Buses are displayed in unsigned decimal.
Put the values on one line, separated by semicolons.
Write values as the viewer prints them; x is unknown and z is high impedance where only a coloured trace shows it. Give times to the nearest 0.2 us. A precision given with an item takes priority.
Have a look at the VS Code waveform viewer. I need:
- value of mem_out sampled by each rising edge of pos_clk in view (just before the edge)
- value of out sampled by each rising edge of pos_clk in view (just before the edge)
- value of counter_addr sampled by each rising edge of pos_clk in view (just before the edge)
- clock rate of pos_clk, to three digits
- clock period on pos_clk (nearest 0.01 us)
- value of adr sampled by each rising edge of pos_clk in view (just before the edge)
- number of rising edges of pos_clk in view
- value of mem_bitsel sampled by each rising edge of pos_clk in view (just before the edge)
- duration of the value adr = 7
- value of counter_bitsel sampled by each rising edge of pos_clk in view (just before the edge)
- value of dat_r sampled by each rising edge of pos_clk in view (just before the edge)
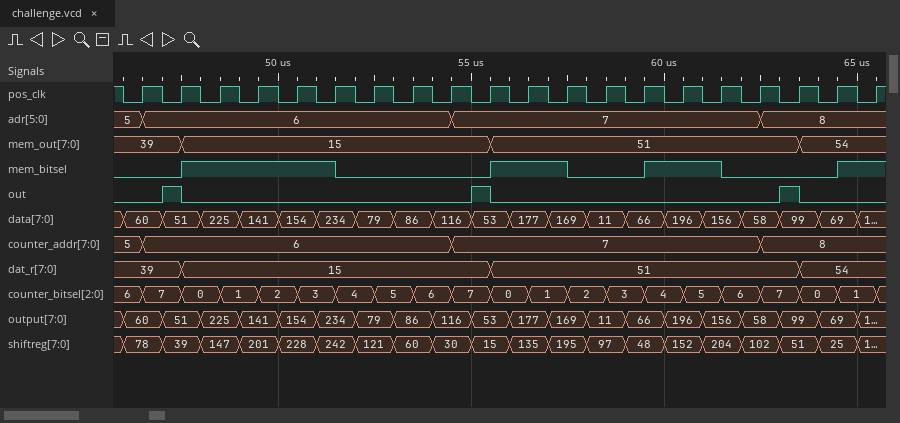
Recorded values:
39, 39, 15, 15, 15, 15, 15, 15, 15, 15, 51, 51, 51, 51, 51, 51, 51, 51, 54, 54; 0 1 0 0 0 0 0 0 0 1 0 0 0 0 0 0 0 1 0 0; 5, 6, 6, 6, 6, 6, 6, 6, 6, 7, 7, 7, 7, 7, 7, 7, 7, 8, 8, 8; 1.00 MHz; 1 us; 5, 6, 6, 6, 6, 6, 6, 6, 6, 7, 7, 7, 7, 7, 7, 7, 7, 8, 8, 8; 20; 0 0 1 1 1 1 0 0 0 0 1 1 0 0 1 1 0 0 0 1; 8 us; 6, 7, 0, 1, 2, 3, 4, 5, 6, 7, 0, 1, 2, 3, 4, 5, 6, 7, 0, 1; 39, 39, 15, 15, 15, 15, 15, 15, 15, 15, 51, 51, 51, 51, 51, 51, 51, 51, 54, 54
